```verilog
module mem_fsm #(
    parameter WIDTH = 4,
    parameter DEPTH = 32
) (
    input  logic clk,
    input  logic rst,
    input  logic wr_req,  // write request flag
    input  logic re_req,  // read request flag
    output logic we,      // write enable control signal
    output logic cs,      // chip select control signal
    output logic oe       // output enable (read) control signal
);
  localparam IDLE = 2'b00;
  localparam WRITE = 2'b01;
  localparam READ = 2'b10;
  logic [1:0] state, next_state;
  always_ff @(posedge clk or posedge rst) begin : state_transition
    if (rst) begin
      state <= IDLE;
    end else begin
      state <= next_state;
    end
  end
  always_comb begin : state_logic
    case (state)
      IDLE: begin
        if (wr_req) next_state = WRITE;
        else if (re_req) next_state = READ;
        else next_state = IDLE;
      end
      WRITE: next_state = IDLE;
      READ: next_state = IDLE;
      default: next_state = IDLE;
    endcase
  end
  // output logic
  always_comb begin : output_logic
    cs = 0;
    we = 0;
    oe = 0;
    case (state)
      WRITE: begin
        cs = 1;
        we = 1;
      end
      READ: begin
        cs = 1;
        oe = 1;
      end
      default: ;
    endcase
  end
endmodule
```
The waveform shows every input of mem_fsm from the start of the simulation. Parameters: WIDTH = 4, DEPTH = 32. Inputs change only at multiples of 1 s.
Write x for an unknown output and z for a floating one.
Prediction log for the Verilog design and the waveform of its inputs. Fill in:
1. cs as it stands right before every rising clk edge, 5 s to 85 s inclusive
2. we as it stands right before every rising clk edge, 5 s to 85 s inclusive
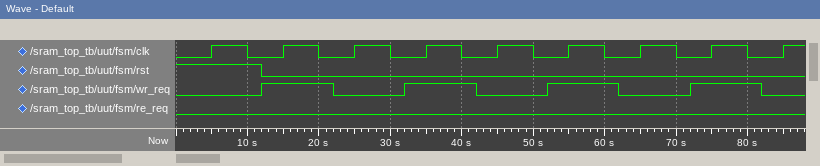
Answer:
0 0 1 0 1 0 1 0 1
0 0 1 0 1 0 1 0 1
